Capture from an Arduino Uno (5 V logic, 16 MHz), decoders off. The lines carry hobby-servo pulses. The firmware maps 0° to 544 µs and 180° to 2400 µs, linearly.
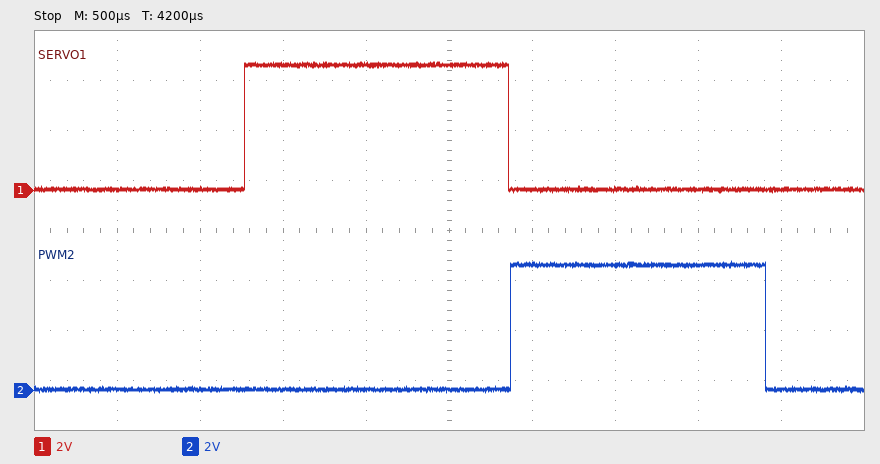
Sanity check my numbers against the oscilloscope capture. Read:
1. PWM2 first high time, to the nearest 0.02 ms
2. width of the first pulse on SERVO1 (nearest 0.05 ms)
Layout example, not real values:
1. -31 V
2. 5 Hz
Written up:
1. 1.54 ms
2. 1.60 ms
